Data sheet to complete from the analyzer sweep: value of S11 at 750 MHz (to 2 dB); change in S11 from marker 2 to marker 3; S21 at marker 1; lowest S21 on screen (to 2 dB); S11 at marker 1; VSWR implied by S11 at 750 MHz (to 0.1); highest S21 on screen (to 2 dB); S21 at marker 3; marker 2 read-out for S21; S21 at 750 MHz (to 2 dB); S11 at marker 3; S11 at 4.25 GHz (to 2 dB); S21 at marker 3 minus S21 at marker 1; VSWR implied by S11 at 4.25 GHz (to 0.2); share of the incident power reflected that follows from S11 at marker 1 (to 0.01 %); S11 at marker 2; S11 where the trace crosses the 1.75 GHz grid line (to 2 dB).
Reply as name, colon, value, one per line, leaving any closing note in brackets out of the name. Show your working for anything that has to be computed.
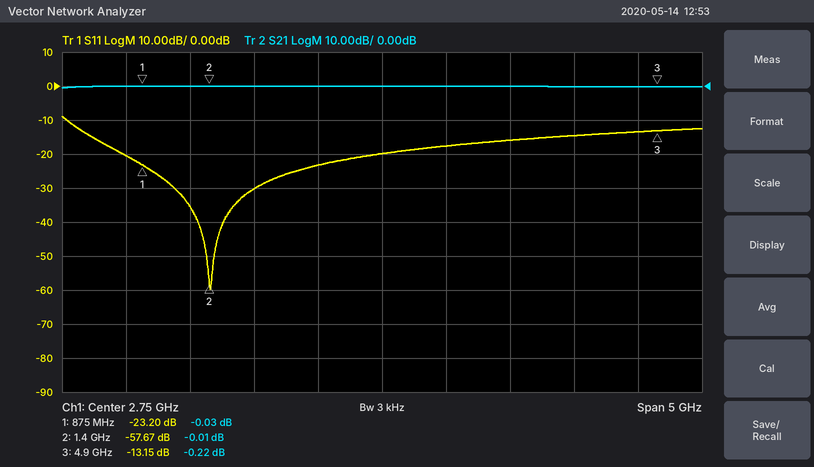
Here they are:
value of S11 at 750 MHz: -20 dB
change in S11 from marker 2 to marker 3: -13.15 − (-57.67) = 44.52 dB
S21 at marker 1: -0.03 dB
lowest S21 on screen: 0 dB
S11 at marker 1: -23.20 dB
VSWR implied by S11 at 750 MHz: |Γ| = 10^(-20/20) = 0.1000; VSWR = (1 + 0.1000)/(1 − 0.1000) ≈ 1.2
highest S21 on screen: 0 dB
S21 at marker 3: -0.22 dB
marker 2 read-out for S21: -0.01 dB
S21 at 750 MHz: 0 dB
S11 at marker 3: -13.15 dB
S11 at 4.25 GHz: -14 dB
S21 at marker 3 minus S21 at marker 1: -0.22 − (-0.03) = -0.19 dB
VSWR implied by S11 at 4.25 GHz: |Γ| = 10^(-14/20) = 0.1995; VSWR = (1 + 0.1995)/(1 − 0.1995) ≈ 1.50, so 1.4 to the nearest 0.2
share of the incident power reflected that follows from S11 at marker 1: 10^(-23.2/10) ≈ 0.48 %
S11 at marker 2: -57.67 dB
S11 where the trace crosses the 1.75 GHz grid line: -30 dB
